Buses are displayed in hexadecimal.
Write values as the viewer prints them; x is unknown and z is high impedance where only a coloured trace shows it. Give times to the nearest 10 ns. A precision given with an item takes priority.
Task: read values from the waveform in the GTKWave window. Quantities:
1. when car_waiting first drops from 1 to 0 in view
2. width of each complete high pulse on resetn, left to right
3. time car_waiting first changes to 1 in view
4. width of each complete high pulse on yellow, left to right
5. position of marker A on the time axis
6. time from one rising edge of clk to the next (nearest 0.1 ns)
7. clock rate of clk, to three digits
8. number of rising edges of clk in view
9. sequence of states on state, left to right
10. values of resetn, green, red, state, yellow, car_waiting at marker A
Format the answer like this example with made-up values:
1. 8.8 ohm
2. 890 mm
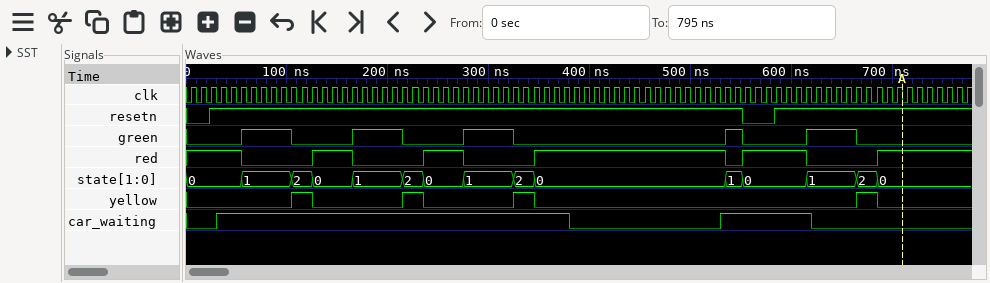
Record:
1. 380 ns
2. 530 ns
3. 30 ns
4. 20 ns, 20 ns, 20 ns, 20 ns
5. 710 ns
6. 10 ns
7. 100 MHz
8. 78
9. 0, 1, 2, 0, 1, 2, 0, 1, 2, 0, 1, 0, 1, 2, 0
10. resetn=1, green=0, red=1, state=0, yellow=0, car_waiting=0
